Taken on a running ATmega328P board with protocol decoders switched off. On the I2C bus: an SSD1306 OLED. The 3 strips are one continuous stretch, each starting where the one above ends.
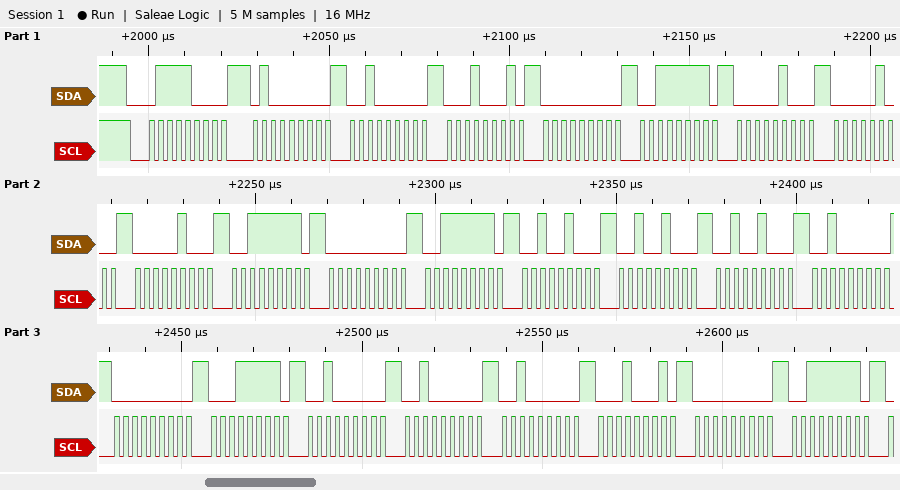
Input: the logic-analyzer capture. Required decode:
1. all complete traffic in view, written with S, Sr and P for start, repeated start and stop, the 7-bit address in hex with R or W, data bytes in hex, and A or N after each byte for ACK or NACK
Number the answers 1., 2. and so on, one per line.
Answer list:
1. S 3CW A 40 A 20 A 11 A 00 A 3F A 04 A 04 A 04 A 3F A 00 A 3F A 24 A 24 A 24 A 20 A 00 A 1F A 20 A 20 A 20 A 11 A 00 A 3F A
